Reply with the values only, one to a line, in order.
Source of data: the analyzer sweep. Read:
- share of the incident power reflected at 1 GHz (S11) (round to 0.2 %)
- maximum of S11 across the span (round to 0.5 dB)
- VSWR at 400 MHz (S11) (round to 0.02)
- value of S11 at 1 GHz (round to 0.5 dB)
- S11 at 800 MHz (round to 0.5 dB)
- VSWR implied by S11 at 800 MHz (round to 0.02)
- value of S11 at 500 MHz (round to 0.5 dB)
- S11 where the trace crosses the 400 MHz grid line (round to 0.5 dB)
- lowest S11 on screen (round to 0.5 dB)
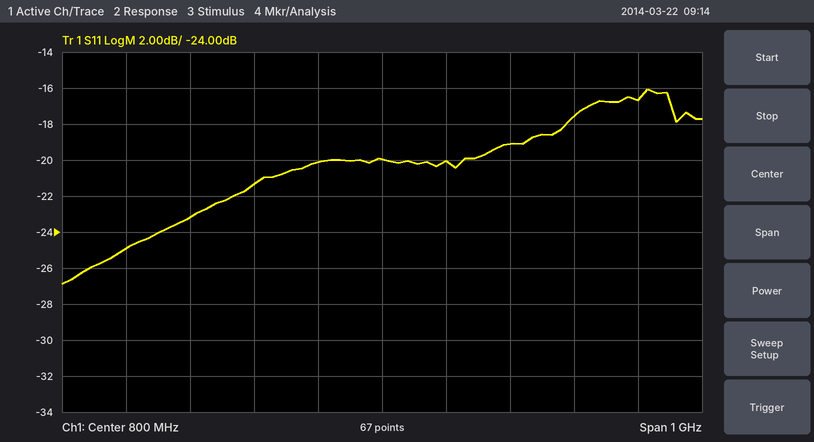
1.2 %
-16.0 dB
1.12
-19.0 dB
-20.0 dB
1.22
-23.0 dB
-25.0 dB
-27.0 dB
